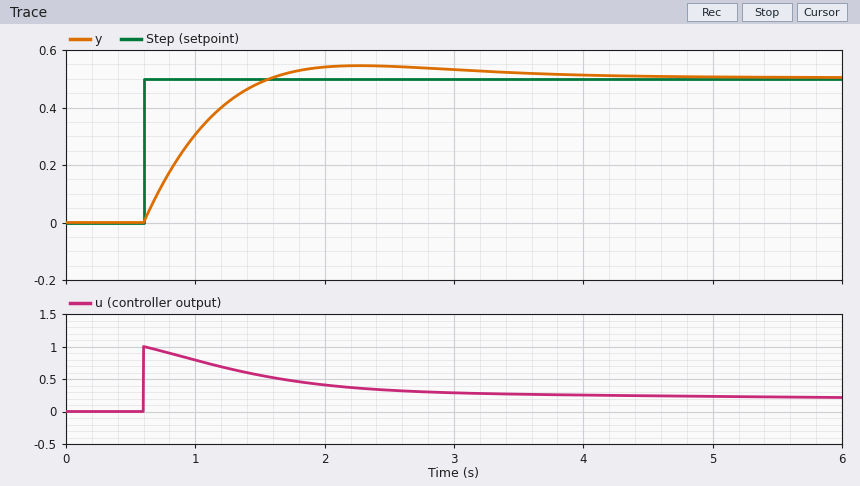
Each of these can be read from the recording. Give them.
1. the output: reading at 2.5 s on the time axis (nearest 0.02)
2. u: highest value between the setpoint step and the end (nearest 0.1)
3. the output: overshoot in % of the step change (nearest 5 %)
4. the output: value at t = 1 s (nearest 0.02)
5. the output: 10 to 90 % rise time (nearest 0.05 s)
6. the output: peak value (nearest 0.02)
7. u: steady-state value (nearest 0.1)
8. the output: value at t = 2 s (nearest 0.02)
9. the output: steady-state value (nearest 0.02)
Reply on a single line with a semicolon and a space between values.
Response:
0.54; 1.0; 10 %; 0.30; 0.70 s; 0.54; 0.2; 0.54; 0.50
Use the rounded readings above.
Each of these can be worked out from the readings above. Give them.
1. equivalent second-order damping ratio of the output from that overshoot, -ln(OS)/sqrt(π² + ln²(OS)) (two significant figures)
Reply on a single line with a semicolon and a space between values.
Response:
0.59
